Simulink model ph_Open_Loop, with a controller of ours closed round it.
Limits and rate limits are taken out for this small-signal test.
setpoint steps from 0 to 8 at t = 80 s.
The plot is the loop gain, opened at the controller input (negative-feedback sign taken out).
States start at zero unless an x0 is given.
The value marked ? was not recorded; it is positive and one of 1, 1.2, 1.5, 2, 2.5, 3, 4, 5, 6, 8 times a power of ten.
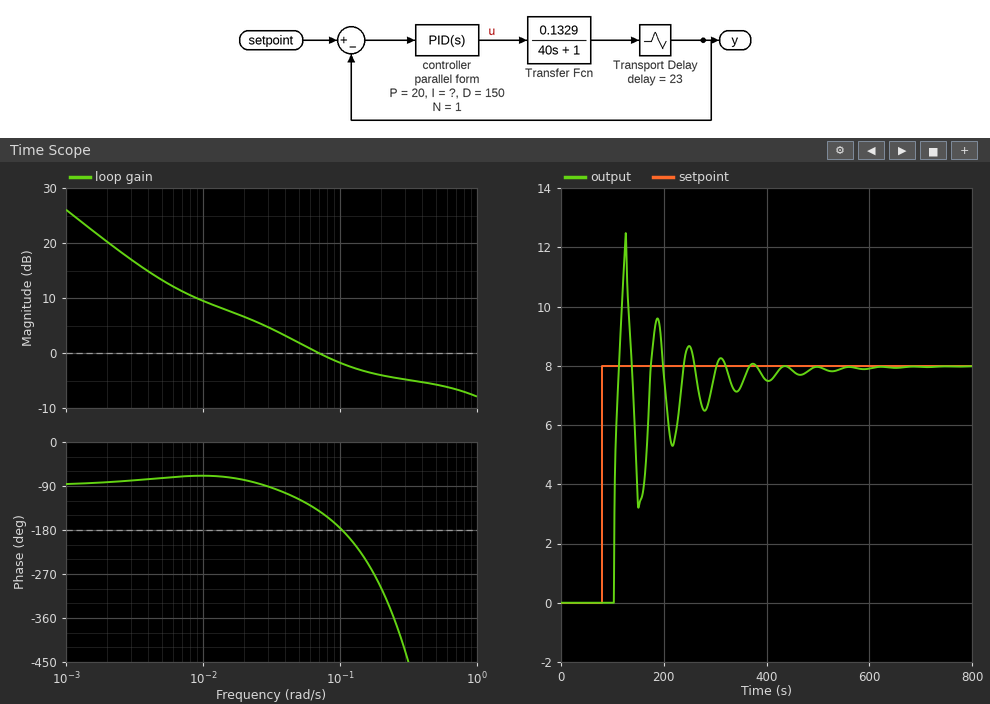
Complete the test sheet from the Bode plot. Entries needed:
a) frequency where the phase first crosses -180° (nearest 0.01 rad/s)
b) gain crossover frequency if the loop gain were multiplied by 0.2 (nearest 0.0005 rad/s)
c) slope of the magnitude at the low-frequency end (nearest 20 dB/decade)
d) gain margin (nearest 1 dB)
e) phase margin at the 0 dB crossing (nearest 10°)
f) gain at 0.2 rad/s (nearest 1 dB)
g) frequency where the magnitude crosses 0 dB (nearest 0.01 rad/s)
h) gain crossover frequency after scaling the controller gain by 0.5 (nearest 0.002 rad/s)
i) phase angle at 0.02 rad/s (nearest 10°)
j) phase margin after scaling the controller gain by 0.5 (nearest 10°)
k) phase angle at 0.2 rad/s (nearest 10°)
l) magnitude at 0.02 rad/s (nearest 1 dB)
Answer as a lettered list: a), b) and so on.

a) 0.10 rad/s
b) 0.0045 rad/s
c) -20 dB/decade
d) 2 dB
e) 40°
f) -4 dB
g) 0.07 rad/s
h) 0.022 rad/s
i) -80°
j) 100°
k) -300°
l) 7 dB
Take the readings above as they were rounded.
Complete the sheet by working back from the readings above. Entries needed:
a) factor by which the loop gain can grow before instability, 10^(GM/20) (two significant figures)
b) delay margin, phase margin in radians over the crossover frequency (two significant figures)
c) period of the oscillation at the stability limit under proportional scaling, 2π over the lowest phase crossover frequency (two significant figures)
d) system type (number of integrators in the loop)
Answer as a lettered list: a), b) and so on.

a) 1.3
b) 10.0 s
c) 63 s
d) 1
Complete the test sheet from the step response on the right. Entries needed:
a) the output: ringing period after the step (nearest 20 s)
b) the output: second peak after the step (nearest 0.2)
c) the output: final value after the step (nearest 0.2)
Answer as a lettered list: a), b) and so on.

a) 60 s
b) 9.6
c) 8.0
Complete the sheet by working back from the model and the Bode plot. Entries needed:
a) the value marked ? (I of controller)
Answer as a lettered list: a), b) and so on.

a) 0.15
